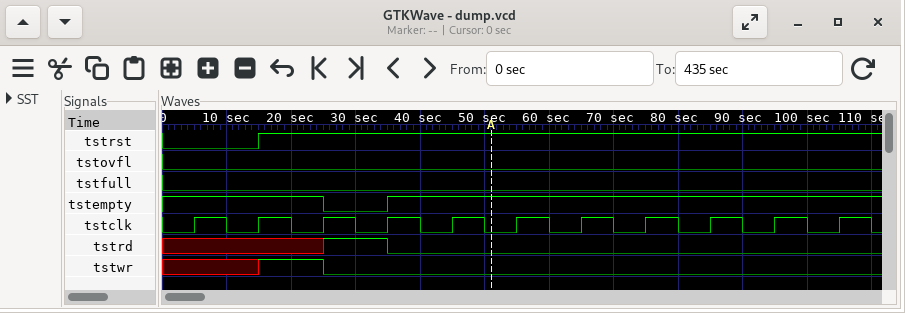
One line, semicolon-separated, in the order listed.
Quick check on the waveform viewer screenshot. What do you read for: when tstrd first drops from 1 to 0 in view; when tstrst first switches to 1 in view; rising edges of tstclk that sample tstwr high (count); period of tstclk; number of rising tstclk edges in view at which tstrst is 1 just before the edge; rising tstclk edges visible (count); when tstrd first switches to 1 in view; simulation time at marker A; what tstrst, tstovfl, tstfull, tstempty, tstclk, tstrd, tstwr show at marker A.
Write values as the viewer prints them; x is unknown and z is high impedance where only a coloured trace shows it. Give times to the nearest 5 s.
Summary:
35 s; 15 s; 1; 10 s; 9; 11; 25 s; 50 s; tstrst=1, tstovfl=0, tstfull=0, tstempty=1, tstclk=0, tstrd=0, tstwr=0
